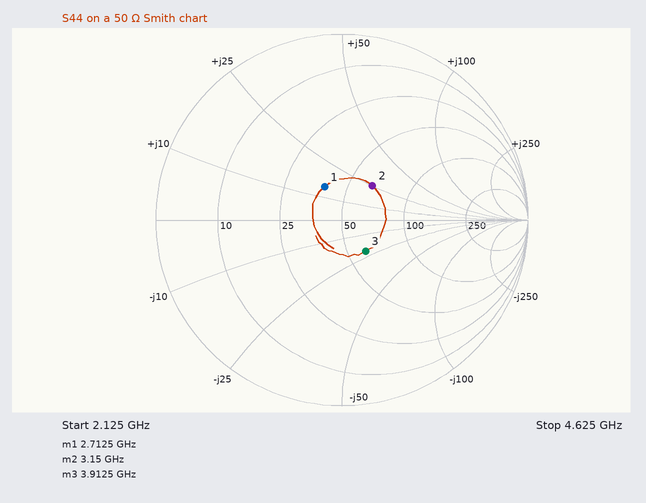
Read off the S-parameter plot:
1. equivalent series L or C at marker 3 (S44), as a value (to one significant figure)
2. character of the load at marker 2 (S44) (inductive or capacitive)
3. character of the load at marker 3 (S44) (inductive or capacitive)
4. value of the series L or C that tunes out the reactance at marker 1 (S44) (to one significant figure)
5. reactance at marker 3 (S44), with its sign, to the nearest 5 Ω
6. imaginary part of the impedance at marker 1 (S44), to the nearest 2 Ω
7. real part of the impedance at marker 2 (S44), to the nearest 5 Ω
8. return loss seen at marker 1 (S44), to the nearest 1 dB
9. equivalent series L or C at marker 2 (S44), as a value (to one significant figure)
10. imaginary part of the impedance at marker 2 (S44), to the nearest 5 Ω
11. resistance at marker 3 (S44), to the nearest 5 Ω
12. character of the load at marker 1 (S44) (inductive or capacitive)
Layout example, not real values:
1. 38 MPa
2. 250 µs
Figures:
1. 2 pF
2. inductive
3. capacitive
4. 4 pF
5. -20 Ω
6. +14 Ω
7. 65 Ω
8. 14 dB
9. 1 nH
10. +25 Ω
11. 60 Ω
12. inductive
